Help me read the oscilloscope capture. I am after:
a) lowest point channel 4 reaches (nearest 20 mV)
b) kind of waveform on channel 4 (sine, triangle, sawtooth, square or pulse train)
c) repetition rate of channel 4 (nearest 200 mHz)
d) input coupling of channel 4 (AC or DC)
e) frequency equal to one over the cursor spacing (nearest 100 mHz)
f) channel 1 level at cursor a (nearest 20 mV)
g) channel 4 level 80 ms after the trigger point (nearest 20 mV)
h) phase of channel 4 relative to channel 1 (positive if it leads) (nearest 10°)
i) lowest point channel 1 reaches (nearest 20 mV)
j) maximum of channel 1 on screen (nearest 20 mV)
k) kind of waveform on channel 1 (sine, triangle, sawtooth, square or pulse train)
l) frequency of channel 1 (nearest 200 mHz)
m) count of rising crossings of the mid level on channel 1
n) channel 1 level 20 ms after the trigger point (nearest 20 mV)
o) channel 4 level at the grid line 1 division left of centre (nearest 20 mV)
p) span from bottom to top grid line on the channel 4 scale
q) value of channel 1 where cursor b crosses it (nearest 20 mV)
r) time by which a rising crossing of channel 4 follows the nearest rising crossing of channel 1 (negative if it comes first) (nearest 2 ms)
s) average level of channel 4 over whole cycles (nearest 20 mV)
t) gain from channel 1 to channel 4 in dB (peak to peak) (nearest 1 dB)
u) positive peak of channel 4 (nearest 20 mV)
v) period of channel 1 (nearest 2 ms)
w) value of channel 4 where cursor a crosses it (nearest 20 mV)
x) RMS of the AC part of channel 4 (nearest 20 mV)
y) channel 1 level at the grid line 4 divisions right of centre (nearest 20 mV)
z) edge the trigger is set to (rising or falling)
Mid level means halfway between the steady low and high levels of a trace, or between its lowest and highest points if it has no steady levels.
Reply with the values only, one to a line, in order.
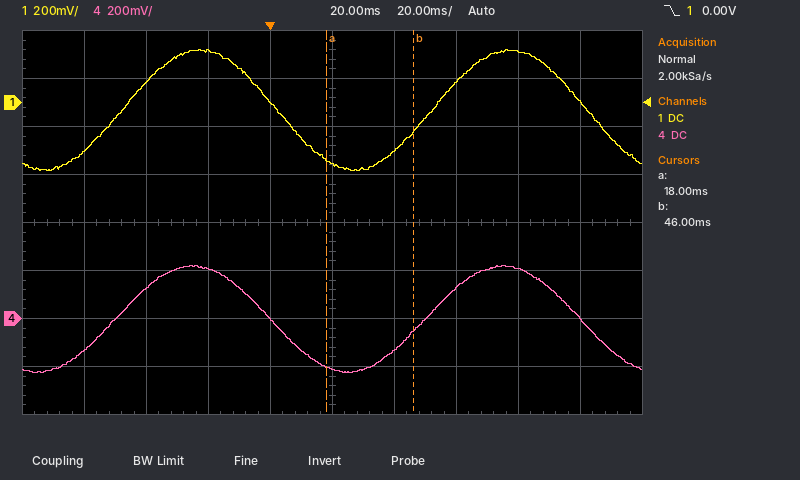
-220 mV
sine
10.0 Hz
DC
35.7 Hz
-240 mV
200 mV
+10°
-280 mV
220 mV
sine
10.0 Hz
2
-260 mV
0 mV
1.6 V
-120 mV
-2 ms
0 mV
-1 dB
220 mV
100 ms
-200 mV
160 mV
0 mV
falling
